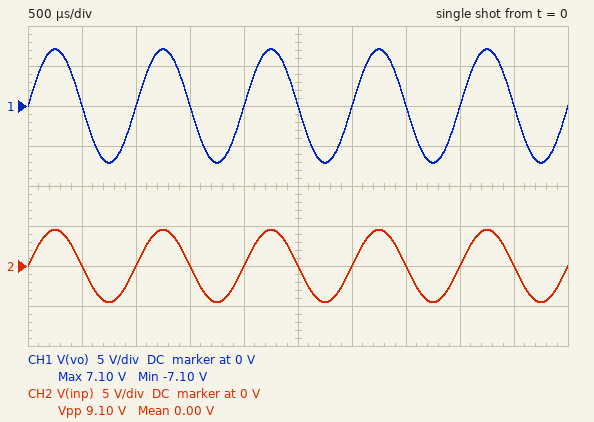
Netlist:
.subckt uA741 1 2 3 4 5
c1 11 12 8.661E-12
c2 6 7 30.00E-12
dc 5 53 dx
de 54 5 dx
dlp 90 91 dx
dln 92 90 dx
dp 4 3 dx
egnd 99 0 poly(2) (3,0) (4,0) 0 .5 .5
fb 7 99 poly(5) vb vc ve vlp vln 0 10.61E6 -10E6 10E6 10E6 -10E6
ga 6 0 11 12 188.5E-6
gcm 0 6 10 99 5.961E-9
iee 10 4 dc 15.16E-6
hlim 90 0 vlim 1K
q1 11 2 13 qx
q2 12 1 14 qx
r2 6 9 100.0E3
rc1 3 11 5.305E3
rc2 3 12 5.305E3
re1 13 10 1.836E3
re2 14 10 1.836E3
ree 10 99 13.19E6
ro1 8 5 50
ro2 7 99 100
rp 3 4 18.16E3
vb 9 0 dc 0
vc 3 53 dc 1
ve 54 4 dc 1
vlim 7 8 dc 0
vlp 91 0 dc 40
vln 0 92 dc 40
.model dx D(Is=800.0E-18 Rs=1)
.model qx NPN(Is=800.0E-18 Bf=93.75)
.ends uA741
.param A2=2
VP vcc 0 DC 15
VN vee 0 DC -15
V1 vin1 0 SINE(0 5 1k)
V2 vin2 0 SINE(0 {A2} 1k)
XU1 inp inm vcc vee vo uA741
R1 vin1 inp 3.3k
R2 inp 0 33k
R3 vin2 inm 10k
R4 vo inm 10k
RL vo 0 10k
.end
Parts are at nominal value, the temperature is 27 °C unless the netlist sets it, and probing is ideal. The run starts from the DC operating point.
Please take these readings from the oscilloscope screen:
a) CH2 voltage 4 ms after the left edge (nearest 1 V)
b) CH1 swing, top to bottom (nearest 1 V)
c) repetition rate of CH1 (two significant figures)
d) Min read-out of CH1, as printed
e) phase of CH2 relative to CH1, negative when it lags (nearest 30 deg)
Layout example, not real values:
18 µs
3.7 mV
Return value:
0 V
14 V
1.0 kHz
-7.10 V
0 deg
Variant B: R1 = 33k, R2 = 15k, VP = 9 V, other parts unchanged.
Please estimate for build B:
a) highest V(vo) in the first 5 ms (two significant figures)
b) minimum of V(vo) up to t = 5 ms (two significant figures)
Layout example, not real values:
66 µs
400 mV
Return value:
1.1 V
-1.1 V
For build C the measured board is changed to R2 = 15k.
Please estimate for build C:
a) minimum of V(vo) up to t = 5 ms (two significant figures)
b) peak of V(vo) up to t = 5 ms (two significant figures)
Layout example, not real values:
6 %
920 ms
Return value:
-6.2 V
6.2 V
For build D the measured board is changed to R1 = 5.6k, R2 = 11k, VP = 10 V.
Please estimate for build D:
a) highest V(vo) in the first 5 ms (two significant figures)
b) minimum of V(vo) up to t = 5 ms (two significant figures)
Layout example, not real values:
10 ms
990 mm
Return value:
4.6 V
-4.6 V
